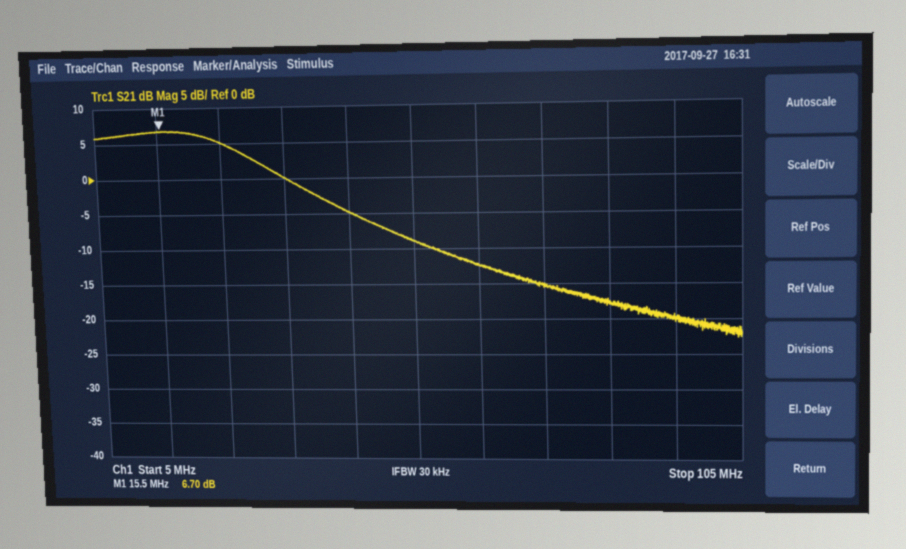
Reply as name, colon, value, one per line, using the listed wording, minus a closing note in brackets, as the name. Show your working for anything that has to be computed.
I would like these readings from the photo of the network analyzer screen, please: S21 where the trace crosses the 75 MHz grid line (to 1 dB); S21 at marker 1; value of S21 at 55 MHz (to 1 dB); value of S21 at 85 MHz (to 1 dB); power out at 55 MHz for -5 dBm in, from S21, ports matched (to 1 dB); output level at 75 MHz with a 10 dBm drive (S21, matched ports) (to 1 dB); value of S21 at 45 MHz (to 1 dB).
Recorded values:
S21 where the trace crosses the 75 MHz grid line: -15 dB
S21 at marker 1: 6.70 dB
value of S21 at 55 MHz: -9 dB
value of S21 at 85 MHz: -18 dB
power out at 55 MHz for -5 dBm in, from S21, ports matched: -5 dBm + (-9 dB) = -14 dBm
output level at 75 MHz with a 10 dBm drive (S21, matched ports): 10 dBm + (-15 dB) = -5 dBm
value of S21 at 45 MHz: -5 dB
